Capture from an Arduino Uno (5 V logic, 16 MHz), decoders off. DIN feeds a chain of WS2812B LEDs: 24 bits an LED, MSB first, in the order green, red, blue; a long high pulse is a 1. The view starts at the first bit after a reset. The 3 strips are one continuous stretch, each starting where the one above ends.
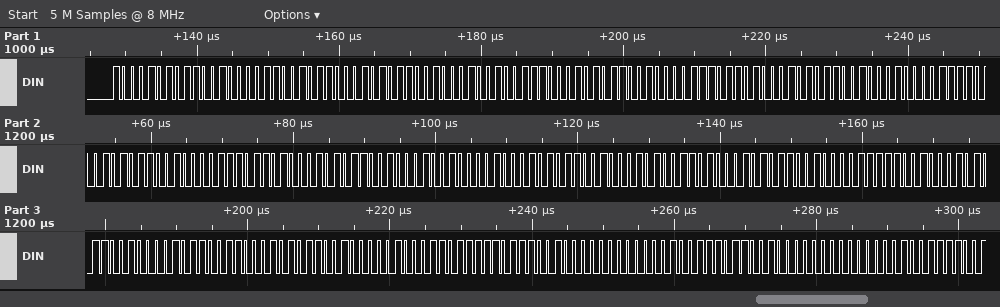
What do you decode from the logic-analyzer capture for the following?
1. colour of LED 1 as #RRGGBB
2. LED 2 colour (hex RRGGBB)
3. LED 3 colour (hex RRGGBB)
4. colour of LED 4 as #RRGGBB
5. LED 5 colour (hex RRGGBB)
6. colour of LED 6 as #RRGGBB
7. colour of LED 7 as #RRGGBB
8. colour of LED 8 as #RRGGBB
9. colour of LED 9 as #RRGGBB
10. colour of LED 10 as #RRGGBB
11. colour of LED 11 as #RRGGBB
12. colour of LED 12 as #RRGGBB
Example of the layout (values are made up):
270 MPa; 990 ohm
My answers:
#C88A65; #C88A93; #C88A76; #C88A87; #C88A76; #C88A90; #C88AA6; #C88A7C; #C88A59; #C88A23; #C87D00; #C84E00
